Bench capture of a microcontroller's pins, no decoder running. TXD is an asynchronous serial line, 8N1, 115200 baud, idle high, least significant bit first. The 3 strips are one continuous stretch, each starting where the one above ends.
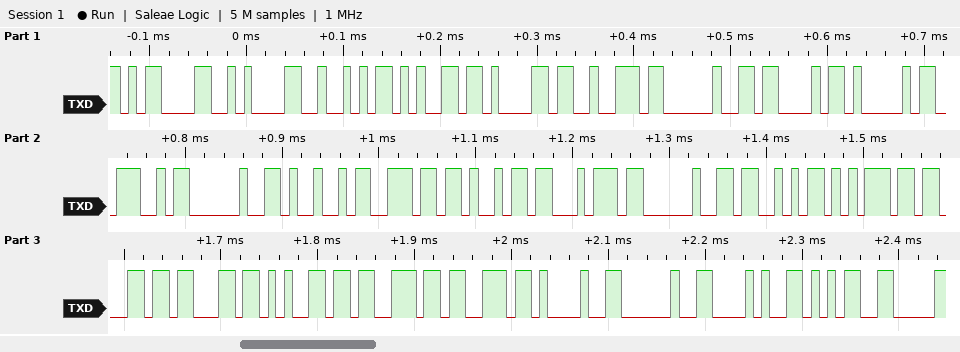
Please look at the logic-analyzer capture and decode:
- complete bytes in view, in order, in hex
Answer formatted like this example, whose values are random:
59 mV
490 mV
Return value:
0D 0A 52 65 61 72 20 43 41 4E 20 49 6E 69 74 20 53 75 63 63 65 73 73 21 20 28 35
